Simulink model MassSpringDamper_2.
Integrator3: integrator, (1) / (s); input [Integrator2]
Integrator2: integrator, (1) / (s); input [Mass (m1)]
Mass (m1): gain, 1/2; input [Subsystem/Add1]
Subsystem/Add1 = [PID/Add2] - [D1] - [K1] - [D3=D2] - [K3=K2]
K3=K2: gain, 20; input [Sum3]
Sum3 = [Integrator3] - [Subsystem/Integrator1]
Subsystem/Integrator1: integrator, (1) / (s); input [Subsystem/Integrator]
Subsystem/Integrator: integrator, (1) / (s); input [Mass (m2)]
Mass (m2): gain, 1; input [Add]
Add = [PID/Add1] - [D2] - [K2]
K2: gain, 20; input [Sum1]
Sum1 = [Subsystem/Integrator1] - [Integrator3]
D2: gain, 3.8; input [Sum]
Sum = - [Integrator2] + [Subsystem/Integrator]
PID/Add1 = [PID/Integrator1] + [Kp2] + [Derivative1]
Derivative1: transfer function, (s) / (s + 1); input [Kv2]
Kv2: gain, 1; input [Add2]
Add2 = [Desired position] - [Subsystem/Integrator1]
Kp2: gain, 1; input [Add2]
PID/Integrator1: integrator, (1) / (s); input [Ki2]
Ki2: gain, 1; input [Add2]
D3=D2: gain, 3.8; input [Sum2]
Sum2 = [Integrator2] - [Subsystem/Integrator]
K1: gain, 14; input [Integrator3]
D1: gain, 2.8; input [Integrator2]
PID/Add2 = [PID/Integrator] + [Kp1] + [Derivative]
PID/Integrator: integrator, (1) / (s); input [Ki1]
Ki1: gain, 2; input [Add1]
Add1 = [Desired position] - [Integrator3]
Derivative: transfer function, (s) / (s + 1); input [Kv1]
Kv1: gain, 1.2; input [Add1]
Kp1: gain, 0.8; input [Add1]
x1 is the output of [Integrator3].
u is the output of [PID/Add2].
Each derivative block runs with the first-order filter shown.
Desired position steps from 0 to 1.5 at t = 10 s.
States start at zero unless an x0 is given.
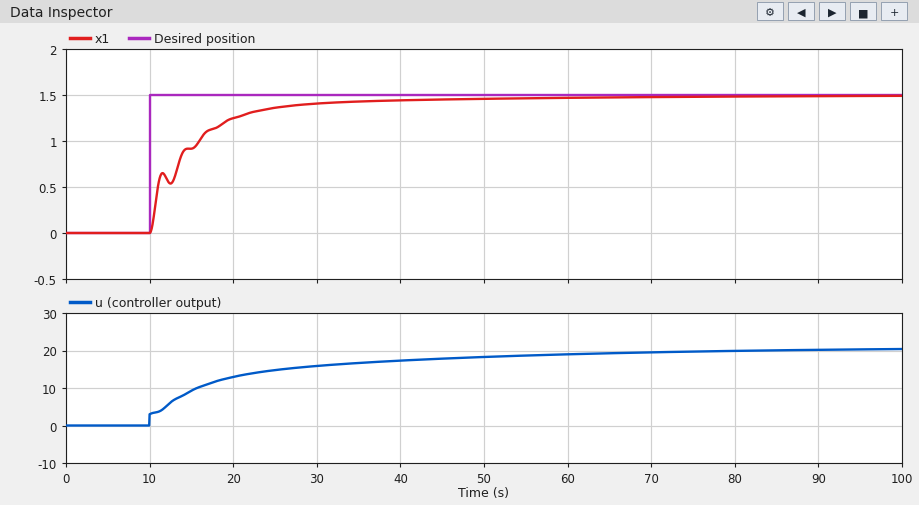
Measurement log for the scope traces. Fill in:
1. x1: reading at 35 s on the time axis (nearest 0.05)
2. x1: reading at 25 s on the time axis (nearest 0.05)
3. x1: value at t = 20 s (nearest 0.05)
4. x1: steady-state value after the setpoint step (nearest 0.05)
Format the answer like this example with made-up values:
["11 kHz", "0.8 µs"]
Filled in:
["1.45", "1.35", "1.25", "1.50"]
